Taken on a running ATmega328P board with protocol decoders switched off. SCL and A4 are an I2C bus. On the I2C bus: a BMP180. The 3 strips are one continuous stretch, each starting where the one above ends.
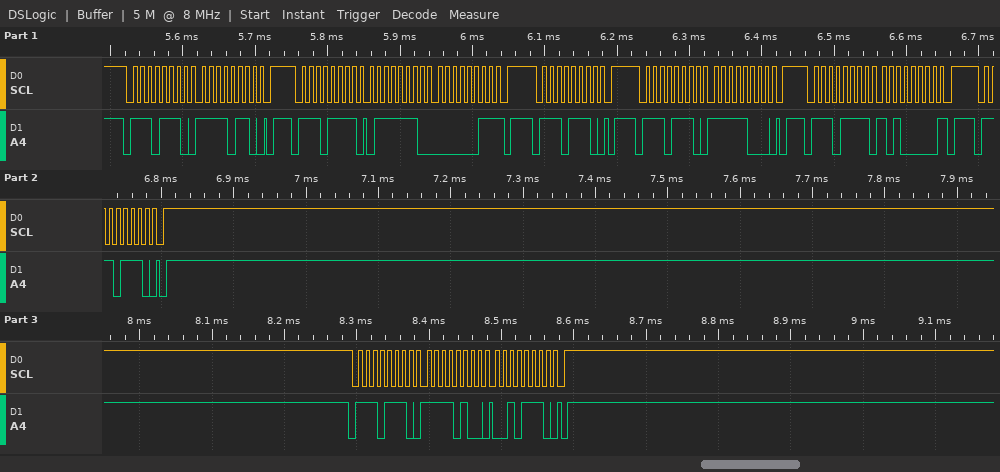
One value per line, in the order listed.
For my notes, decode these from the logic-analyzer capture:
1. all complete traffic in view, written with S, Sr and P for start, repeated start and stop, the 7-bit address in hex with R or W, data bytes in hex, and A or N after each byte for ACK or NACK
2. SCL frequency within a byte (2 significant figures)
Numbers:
S 77W A F6 A P S 77R A 7E A 03 N P S 77W A P S 77W A F8 A P S 77R A A0 N P S 77W A P S 77W A F4 A 2E A P
100 kHz
